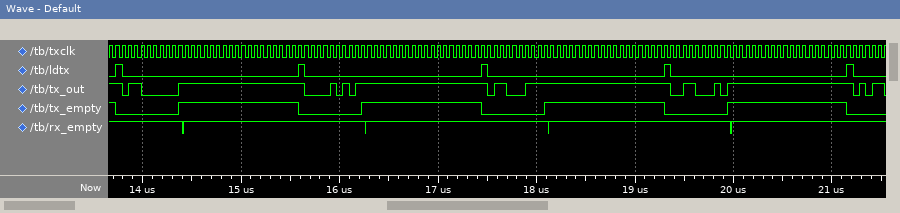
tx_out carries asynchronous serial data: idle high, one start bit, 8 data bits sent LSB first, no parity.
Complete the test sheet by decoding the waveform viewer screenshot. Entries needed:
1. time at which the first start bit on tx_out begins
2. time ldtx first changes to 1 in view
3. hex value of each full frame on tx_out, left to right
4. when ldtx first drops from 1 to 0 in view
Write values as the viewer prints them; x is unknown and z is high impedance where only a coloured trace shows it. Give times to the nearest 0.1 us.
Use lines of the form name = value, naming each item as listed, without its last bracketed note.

time at which the first start bit on tx_out begins = 13.8 us
time ldtx first changes to 1 in view = 13.7 us
hex value of each full frame on tx_out, left to right = 03, A8, E3, 46
when ldtx first drops from 1 to 0 in view = 13.8 us
